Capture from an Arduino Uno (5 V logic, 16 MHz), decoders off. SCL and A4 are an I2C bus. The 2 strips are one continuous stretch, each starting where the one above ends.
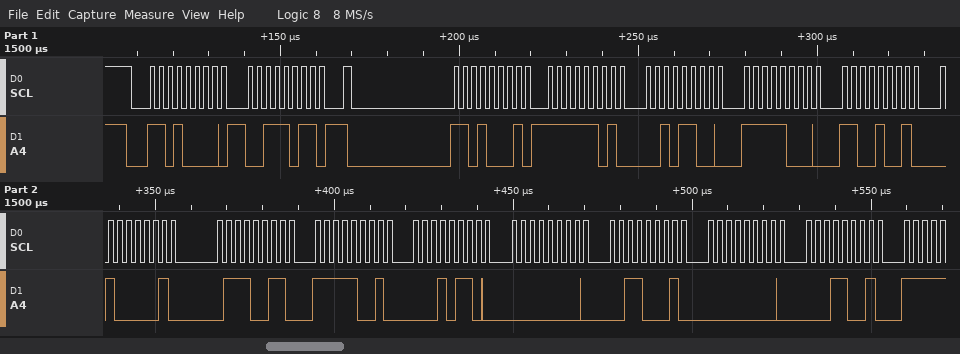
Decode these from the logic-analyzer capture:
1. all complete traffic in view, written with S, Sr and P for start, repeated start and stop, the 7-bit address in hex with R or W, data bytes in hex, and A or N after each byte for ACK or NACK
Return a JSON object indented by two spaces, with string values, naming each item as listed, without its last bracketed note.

{
  "all complete traffic in view, written with S, Sr and P for start, repeated start and stop, the 7-bit address in hex with R or W, data bytes in hex, and A or N after each byte for ACK or NACK": "S 68W A 3B A Sr 68R A FD A 2C A F8 A C9 A 41 A 73 A F9 A 16 A 00 A 31 A 00 A 19 A"
}
